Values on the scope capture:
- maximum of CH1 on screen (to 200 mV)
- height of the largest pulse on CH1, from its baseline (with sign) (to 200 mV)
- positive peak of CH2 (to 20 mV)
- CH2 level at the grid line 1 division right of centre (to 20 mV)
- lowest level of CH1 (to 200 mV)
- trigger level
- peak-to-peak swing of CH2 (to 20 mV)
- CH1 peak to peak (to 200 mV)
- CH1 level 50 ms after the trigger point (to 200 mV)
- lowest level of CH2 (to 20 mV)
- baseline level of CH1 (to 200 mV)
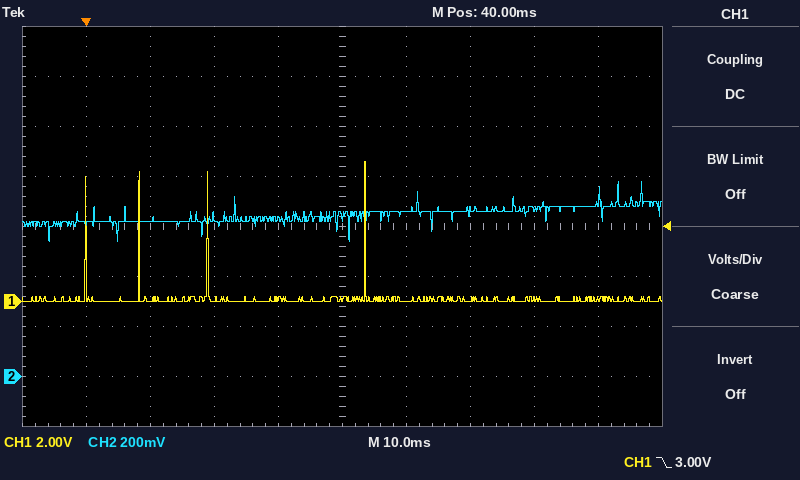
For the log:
5.6 V
+5.6 V
780 mV
660 mV
0.0 V
3.00 V
240 mV
5.6 V
0.0 V
540 mV
0.0 V
